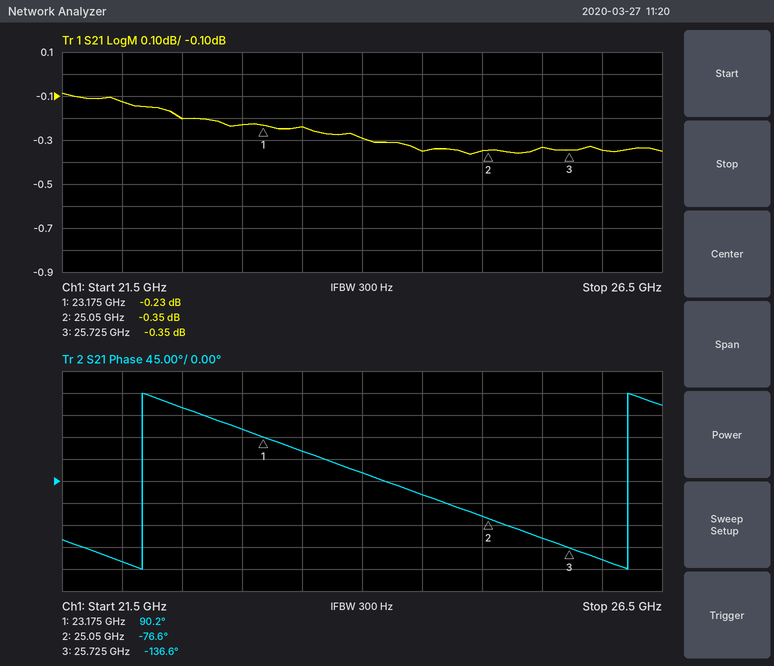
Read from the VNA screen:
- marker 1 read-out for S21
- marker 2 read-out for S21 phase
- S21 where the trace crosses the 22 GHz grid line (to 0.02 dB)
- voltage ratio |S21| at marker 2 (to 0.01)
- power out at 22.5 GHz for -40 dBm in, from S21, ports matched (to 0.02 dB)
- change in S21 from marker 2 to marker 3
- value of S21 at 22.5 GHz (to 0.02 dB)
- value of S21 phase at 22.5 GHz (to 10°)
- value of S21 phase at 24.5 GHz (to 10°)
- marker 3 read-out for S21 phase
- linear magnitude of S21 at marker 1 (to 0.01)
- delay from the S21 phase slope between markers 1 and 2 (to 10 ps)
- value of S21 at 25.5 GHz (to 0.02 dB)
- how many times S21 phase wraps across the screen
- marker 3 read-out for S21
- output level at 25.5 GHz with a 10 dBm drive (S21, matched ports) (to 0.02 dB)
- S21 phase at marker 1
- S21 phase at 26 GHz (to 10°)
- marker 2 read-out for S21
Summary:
-0.23 dB
-76.6°
-0.12 dB
0.96
-40.20 dBm
0.00 dB
-0.20 dB
150°
-30°
-136.6°
0.97
250 ps
-0.34 dB
2
-0.35 dB
9.66 dBm
90.2°
-160°
-0.35 dB
